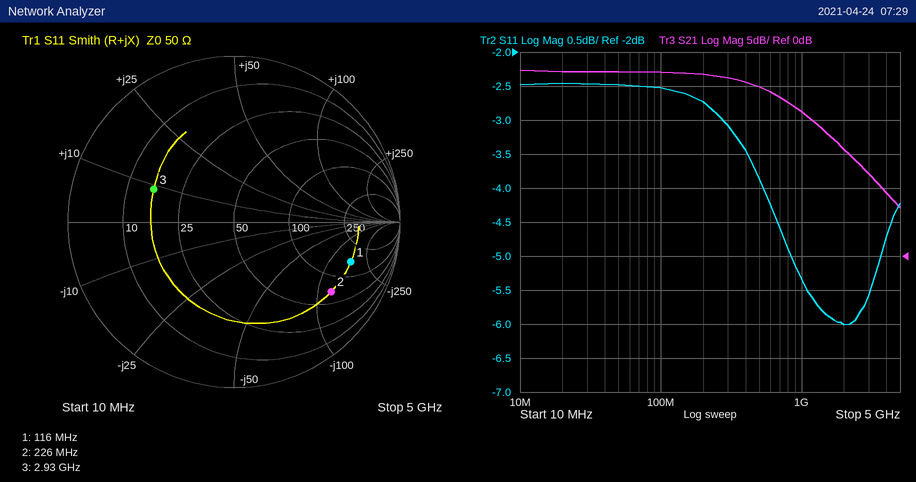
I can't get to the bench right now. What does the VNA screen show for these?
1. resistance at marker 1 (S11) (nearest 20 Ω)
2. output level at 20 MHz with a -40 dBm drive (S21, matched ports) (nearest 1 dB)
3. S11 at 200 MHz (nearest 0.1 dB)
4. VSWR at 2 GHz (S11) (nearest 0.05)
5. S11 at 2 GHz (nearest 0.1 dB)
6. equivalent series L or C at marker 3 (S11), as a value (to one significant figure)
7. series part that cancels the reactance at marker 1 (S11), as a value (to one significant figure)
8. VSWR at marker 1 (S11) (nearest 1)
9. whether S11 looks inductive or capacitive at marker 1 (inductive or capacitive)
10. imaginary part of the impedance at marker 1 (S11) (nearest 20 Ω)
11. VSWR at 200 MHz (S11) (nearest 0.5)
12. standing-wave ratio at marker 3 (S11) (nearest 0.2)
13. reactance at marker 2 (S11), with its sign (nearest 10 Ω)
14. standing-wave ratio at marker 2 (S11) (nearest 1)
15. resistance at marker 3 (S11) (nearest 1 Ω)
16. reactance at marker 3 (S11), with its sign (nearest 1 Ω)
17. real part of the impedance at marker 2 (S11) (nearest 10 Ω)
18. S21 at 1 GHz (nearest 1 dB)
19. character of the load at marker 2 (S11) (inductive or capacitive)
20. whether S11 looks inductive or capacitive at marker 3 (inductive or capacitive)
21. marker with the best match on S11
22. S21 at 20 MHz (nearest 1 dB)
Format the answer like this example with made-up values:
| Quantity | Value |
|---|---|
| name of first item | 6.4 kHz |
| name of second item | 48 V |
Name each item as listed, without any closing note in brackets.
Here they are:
| Quantity | Value |
|---|---|
| resistance at marker 1 (S11) | 160 Ω |
| output level at 20 MHz with a -40 dBm drive (S21, matched ports) | -13 dBm |
| S11 at 200 MHz | -2.7 dB |
| VSWR at 2 GHz (S11) | 3.00 |
| S11 at 2 GHz | -6.0 dB |
| equivalent series L or C at marker 3 (S11), as a value | 500 pH |
| series part that cancels the reactance at marker 1 (S11), as a value | 200 nH |
| VSWR at marker 1 (S11) | 7 |
| whether S11 looks inductive or capacitive at marker 1 | capacitive |
| imaginary part of the impedance at marker 1 (S11) | -160 Ω |
| VSWR at 200 MHz (S11) | 6.5 |
| standing-wave ratio at marker 3 (S11) | 3.2 |
| reactance at marker 2 (S11), with its sign | -120 Ω |
| standing-wave ratio at marker 2 (S11) | 6 |
| resistance at marker 3 (S11) | 16 Ω |
| reactance at marker 3 (S11), with its sign | +9 Ω |
| real part of the impedance at marker 2 (S11) | 70 Ω |
| S21 at 1 GHz | 21 dB |
| character of the load at marker 2 (S11) | capacitive |
| whether S11 looks inductive or capacitive at marker 3 | inductive |
| marker with the best match on S11 | marker 3 |
| S21 at 20 MHz | 27 dB |
